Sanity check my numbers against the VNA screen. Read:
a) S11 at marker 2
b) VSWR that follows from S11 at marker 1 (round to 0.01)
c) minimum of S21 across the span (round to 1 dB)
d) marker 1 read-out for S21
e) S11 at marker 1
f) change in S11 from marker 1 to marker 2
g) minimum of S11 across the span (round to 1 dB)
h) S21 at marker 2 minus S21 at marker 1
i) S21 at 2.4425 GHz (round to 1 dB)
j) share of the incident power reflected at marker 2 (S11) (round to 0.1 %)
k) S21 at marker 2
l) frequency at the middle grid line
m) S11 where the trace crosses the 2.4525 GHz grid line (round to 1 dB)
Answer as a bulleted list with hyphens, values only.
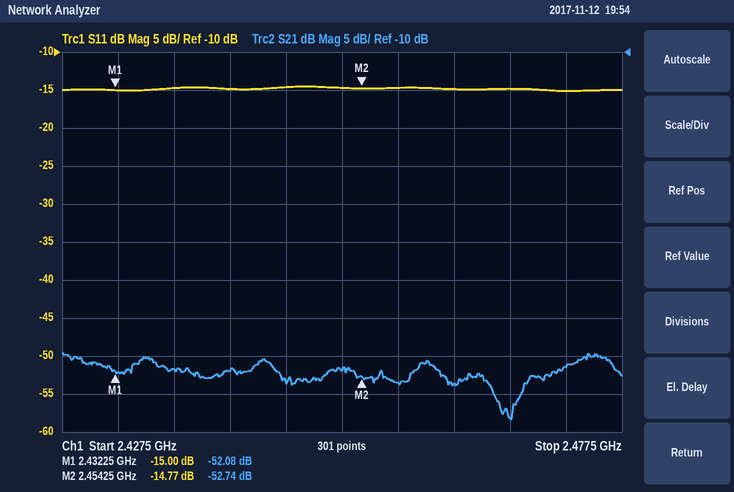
- -14.77 dB
- 1.43
- -58 dB
- -52.08 dB
- -15.00 dB
- 0.23 dB
- -15 dB
- -0.66 dB
- -52 dB
- 3.3 %
- -52.74 dB
- 2.4525 GHz
- -15 dB
